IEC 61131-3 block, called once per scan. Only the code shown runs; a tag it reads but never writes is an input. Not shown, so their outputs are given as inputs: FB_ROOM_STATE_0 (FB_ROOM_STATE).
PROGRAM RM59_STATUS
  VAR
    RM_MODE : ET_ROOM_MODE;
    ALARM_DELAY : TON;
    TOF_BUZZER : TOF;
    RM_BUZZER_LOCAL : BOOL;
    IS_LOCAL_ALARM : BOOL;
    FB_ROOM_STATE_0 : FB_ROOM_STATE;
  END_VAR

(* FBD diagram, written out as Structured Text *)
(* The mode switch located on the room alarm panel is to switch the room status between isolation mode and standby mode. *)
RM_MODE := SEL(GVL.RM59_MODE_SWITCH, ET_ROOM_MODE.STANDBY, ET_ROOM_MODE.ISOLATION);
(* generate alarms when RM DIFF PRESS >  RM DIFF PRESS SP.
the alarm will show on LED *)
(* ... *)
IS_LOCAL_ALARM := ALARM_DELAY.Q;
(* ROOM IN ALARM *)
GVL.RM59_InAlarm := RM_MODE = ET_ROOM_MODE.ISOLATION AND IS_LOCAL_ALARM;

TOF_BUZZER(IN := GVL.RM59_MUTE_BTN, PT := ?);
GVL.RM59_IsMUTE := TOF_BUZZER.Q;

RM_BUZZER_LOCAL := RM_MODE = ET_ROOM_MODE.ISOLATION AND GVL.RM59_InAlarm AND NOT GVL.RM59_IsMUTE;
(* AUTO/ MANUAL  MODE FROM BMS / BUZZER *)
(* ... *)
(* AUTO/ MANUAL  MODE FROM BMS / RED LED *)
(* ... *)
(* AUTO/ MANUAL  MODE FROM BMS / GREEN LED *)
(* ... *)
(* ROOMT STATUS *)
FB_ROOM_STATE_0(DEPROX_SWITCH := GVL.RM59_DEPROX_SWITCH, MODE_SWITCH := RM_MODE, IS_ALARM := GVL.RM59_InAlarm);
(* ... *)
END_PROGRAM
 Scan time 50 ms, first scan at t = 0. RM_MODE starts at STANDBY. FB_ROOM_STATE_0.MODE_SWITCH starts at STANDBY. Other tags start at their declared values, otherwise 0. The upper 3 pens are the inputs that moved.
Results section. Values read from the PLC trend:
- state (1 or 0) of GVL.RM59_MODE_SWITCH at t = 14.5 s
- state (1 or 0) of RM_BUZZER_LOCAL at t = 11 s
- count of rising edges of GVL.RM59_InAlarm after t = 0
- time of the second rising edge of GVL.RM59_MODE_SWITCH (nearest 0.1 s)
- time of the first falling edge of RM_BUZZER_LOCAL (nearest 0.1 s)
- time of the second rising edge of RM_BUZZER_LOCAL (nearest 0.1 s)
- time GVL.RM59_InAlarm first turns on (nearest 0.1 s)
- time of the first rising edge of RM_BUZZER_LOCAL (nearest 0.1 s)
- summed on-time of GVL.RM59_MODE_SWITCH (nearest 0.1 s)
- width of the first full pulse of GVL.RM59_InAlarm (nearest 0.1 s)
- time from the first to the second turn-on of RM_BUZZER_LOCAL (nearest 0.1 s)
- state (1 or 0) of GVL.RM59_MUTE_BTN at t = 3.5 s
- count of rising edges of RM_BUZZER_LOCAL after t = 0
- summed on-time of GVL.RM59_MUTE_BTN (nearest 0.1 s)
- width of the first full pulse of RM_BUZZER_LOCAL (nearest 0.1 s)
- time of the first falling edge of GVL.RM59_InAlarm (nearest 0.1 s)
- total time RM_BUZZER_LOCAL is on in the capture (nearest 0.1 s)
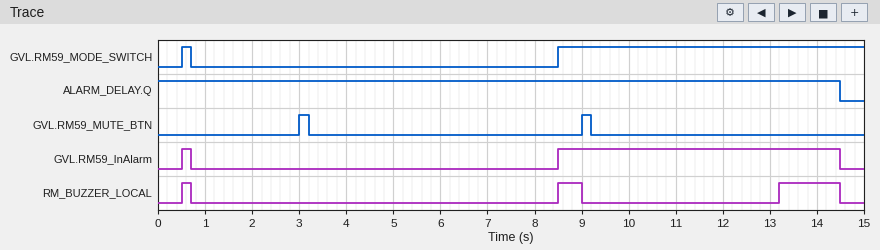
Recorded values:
1
0
2
8.5 s
0.7 s
8.5 s
0.5 s
0.5 s
6.7 s
0.2 s
8.0 s
0
3
0.4 s
0.2 s
0.7 s
2.0 s
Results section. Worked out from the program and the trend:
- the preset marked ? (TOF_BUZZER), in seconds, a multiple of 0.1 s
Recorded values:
4.0 s
